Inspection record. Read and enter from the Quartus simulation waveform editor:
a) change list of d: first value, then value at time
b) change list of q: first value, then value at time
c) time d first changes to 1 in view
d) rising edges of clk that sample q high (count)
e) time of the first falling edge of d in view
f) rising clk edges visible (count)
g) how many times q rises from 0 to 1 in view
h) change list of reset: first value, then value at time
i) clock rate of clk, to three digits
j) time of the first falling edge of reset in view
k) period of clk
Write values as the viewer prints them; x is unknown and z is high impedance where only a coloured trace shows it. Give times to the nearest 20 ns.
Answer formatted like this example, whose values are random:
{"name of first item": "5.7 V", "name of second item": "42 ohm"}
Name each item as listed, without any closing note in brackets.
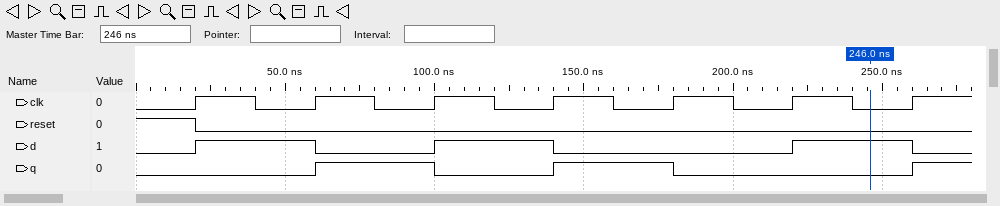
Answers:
{"change list of d: first value, then value at time": "0, 1 at 20 ns, 0 at 60 ns, 1 at 100 ns, 0 at 140 ns, 1 at 220 ns, 0 at 260 ns", "change list of q: first value, then value at time": "0, 1 at 60 ns, 0 at 100 ns, 1 at 140 ns, 0 at 180 ns, 1 at 260 ns", "time d first changes to 1 in view": "20 ns", "rising edges of clk that sample q high": "2", "time of the first falling edge of d in view": "60 ns", "rising clk edges visible": "7", "how many times q rises from 0 to 1 in view": "3", "change list of reset: first value, then value at time": "1, 0 at 20 ns", "clock rate of clk, to three digits": "25.0 MHz", "time of the first falling edge of reset in view": "20 ns", "period of clk": "40 ns"}
